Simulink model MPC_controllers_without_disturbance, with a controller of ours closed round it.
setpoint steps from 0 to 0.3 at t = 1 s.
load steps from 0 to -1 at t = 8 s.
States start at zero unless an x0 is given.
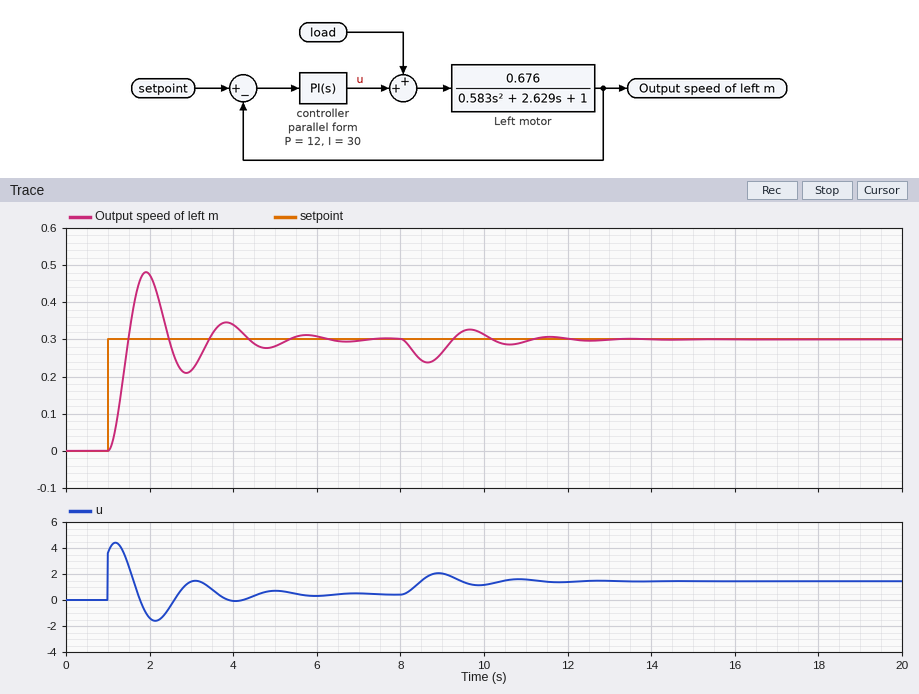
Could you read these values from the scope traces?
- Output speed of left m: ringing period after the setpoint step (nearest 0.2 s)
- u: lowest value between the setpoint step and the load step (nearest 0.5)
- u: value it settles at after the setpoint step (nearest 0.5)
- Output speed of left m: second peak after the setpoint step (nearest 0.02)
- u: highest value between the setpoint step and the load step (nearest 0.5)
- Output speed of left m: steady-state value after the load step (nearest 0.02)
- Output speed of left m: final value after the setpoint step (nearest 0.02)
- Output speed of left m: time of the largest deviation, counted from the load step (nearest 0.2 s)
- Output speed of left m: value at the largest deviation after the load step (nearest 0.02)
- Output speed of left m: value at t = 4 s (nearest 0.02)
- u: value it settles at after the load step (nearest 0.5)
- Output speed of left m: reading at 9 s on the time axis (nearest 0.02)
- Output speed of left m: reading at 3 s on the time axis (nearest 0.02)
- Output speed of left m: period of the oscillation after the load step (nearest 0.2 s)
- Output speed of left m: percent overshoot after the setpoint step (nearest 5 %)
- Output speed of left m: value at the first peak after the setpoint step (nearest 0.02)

2.0 s
-1.5
0.5
0.34
4.5
0.30
0.30
0.6 s
0.24
0.34
1.5
0.26
0.22
2.0 s
60 %
0.48
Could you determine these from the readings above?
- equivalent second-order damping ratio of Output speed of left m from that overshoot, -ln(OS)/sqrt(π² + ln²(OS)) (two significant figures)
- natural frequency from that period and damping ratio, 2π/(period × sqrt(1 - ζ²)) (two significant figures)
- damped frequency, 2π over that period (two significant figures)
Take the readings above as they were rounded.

0.16
3.2 rad/s
3.1 rad/s
